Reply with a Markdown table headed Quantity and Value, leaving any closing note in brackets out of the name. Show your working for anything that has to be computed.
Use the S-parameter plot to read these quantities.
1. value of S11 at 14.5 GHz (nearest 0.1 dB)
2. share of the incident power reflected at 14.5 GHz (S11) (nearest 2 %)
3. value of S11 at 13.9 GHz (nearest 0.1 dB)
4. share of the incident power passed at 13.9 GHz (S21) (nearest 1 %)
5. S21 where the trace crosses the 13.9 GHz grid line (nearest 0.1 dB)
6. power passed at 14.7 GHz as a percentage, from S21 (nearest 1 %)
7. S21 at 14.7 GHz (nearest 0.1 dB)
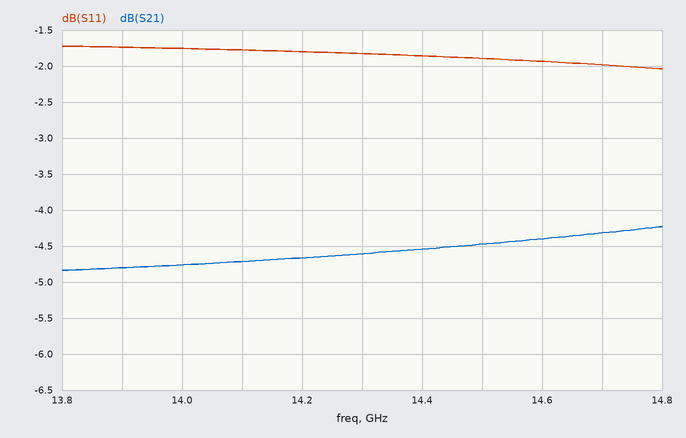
| Quantity | Value |
|---|---|
| value of S11 at 14.5 GHz | -1.9 dB |
| share of the incident power reflected at 14.5 GHz (S11) | 10^(-1.9/10) ≈ 64.6 %, so 64 % to the nearest 2 % |
| value of S11 at 13.9 GHz | -1.7 dB |
| share of the incident power passed at 13.9 GHz (S21) | 10^(-4.8/10) ≈ 33 % |
| S21 where the trace crosses the 13.9 GHz grid line | -4.8 dB |
| power passed at 14.7 GHz as a percentage, from S21 | 10^(-4.3/10) ≈ 37 % |
| S21 at 14.7 GHz | -4.3 dB |
